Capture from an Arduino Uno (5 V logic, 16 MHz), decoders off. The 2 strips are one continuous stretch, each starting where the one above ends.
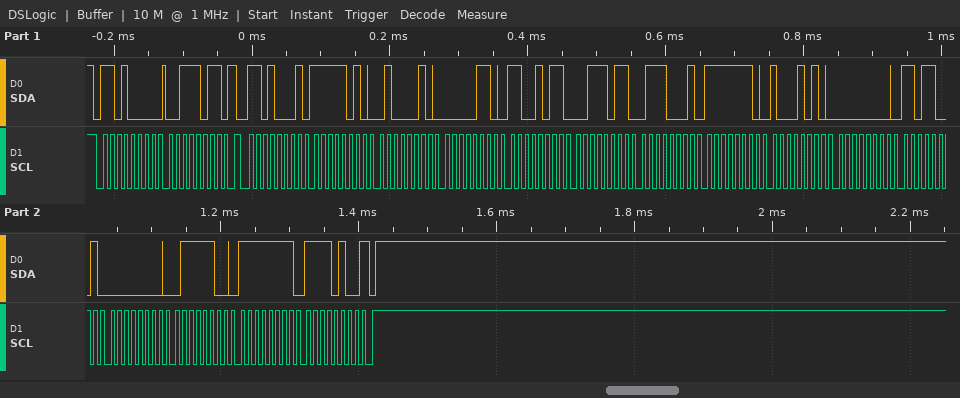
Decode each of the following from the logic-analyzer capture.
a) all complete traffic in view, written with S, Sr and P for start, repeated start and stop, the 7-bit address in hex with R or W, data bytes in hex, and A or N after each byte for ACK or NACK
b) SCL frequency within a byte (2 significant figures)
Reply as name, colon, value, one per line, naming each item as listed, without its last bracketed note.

all complete traffic in view, written with S, Sr and P for start, repeated start and stop, the 7-bit address in hex with R or W, data bytes in hex, and A or N after each byte for ACK or NACK: S 68W A 3B A Sr 68R A FA A 42 A 06 A CB A 3B A 71 A FE A 8A A 00 A D9 A 00 A 7C A FF A F4 N P
SCL frequency within a byte: 100 kHz
